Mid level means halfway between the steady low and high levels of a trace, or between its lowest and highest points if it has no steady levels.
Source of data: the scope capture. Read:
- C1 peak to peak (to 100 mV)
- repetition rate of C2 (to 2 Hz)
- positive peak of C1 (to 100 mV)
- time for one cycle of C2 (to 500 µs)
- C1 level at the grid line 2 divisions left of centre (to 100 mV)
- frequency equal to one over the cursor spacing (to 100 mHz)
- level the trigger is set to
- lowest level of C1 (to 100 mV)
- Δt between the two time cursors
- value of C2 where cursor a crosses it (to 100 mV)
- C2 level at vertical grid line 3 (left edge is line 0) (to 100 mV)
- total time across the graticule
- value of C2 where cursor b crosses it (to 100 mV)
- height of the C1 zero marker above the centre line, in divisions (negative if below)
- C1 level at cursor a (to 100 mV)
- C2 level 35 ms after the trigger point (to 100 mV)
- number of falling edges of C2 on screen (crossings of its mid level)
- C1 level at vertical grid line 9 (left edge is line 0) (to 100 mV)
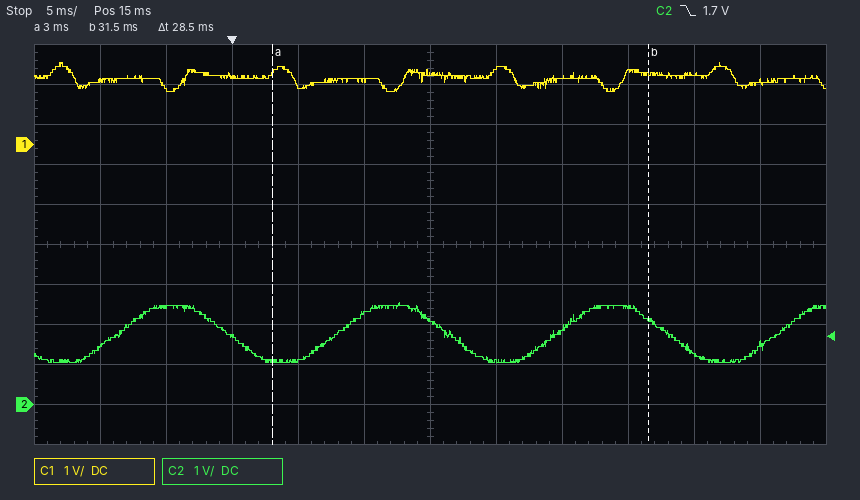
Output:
700 mV
60 Hz
2.0 V
16.5 ms
1.5 V
35.1 Hz
1.7 V
1.3 V
28.5 ms
1.1 V
1.7 V
60 ms
2.1 V
+2.5 div
1.8 V
1.3 V
3
1.8 V
